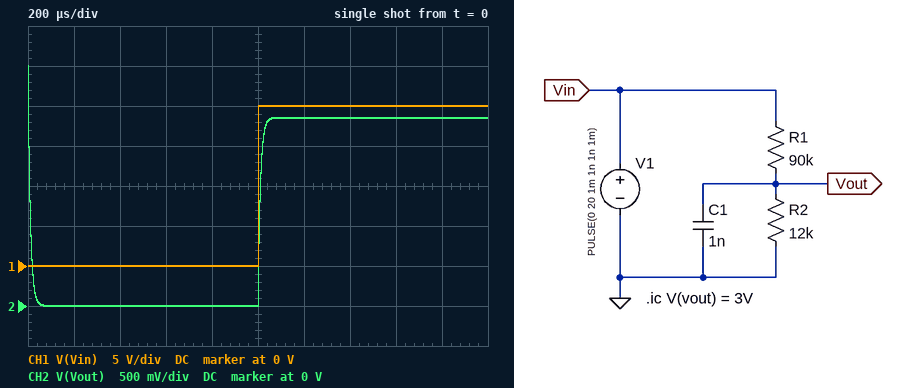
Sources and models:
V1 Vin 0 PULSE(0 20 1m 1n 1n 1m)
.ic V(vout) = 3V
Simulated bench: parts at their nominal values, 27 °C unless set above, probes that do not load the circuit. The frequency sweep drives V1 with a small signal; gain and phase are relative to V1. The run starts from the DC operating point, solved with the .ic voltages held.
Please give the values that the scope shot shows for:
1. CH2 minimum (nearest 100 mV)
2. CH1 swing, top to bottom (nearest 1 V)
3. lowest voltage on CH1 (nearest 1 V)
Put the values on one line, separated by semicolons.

0 V; 20 V; 0 V
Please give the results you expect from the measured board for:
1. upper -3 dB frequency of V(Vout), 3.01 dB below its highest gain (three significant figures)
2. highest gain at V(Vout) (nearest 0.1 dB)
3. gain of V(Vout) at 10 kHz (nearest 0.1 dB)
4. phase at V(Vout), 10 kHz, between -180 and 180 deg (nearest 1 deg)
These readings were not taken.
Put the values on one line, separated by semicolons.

15.0 kHz; -18.6 dB; -20.2 dB; -34 deg
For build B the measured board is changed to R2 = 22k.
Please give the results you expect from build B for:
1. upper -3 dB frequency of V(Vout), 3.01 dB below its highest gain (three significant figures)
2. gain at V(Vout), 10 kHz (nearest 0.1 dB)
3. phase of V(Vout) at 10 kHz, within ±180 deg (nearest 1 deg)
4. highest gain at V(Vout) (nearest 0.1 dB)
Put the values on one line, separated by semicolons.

9.00 kHz; -17.6 dB; -48 deg; -14.1 dB
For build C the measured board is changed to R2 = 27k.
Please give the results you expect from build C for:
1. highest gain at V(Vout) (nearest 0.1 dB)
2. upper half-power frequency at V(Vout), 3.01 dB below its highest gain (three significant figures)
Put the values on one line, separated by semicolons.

-12.7 dB; 7.66 kHz
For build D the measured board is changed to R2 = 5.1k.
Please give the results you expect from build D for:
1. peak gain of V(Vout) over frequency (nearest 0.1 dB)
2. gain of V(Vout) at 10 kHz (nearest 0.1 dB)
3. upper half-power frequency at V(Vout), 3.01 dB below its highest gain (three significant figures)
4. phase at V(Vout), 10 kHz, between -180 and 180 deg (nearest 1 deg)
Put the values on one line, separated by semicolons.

-25.4 dB; -25.8 dB; 33.0 kHz; -17 deg
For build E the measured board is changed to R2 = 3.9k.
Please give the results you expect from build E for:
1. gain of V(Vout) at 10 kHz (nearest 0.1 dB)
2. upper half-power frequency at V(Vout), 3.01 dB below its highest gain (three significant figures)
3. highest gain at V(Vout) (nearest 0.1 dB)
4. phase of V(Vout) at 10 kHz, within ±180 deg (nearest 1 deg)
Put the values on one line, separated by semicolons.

-27.9 dB; 42.6 kHz; -27.6 dB; -13 deg
